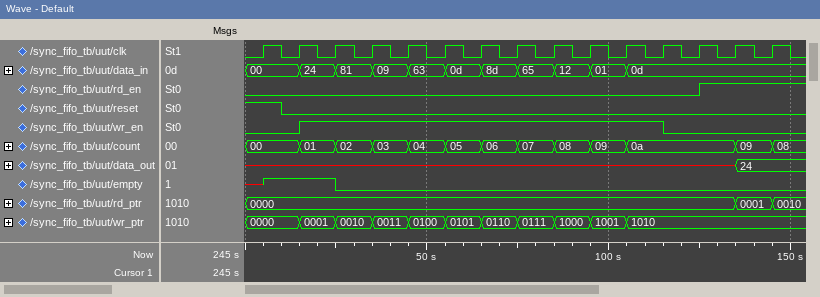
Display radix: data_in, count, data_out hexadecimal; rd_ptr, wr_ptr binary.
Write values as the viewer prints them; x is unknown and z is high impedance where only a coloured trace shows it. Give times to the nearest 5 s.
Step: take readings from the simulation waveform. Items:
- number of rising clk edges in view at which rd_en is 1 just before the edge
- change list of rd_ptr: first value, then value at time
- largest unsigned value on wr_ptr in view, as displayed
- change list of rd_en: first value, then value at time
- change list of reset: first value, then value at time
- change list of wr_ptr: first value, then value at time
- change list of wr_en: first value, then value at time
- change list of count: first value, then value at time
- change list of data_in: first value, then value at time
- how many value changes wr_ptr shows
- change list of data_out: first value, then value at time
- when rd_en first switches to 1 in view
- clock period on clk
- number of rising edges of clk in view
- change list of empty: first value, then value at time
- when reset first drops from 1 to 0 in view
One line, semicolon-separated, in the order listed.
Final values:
2; 0000, 0001 at 135 s, 0010 at 145 s; 1010; 0, 1 at 125 s; 1, 0 at 10 s; 0000, 0001 at 15 s, 0010 at 25 s, 0011 at 35 s, 0100 at 45 s, 0101 at 55 s, 0110 at 65 s, 0111 at 75 s, 1000 at 85 s, 1001 at 95 s, 1010 at 105 s; 0, 1 at 15 s, 0 at 115 s; 00, 01 at 15 s, 02 at 25 s, 03 at 35 s, 04 at 45 s, 05 at 55 s, 06 at 65 s, 07 at 75 s, 08 at 85 s, 09 at 95 s, 0a at 105 s, 09 at 135 s, 08 at 145 s; 00, 24 at 15 s, 81 at 25 s, 09 at 35 s, 63 at 45 s, 0d at 55 s, 8d at 65 s, 65 at 75 s, 12 at 85 s, 01 at 95 s, 0d at 105 s; 10; x, 24 at 135 s; 125 s; 10 s; 15; x, 1 at 5 s, 0 at 25 s; 10 s
